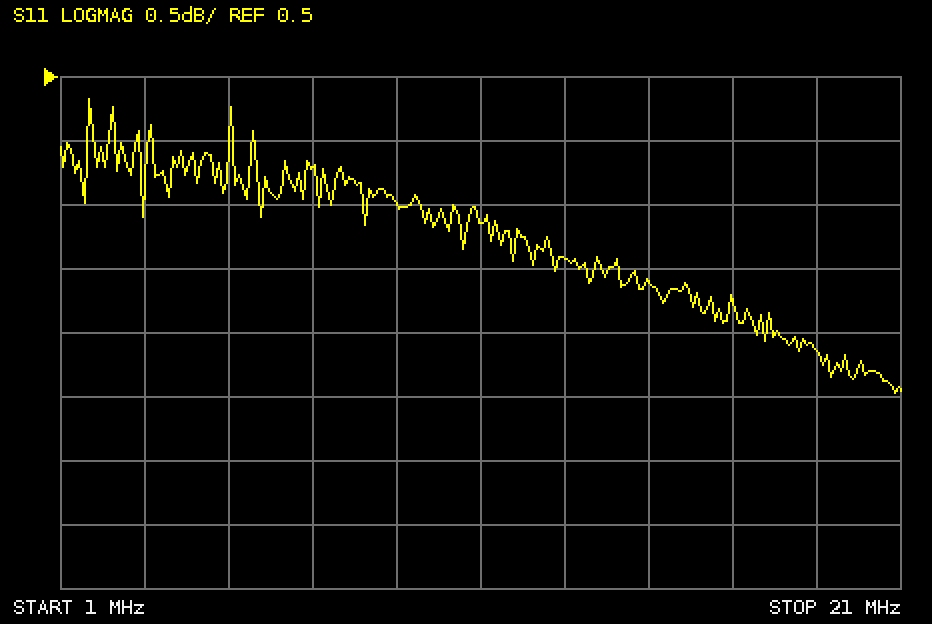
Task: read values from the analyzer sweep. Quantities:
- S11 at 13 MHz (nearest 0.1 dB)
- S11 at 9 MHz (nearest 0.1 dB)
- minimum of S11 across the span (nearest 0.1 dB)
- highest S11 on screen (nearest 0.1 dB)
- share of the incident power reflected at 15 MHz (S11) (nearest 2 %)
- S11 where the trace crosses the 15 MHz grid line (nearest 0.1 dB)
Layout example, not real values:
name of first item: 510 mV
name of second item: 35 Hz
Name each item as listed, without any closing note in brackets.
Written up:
S11 at 13 MHz: -0.9 dB
S11 at 9 MHz: -0.5 dB
minimum of S11 across the span: -2.0 dB
highest S11 on screen: 0.3 dB
share of the incident power reflected at 15 MHz (S11): 78 %
S11 where the trace crosses the 15 MHz grid line: -1.1 dB
